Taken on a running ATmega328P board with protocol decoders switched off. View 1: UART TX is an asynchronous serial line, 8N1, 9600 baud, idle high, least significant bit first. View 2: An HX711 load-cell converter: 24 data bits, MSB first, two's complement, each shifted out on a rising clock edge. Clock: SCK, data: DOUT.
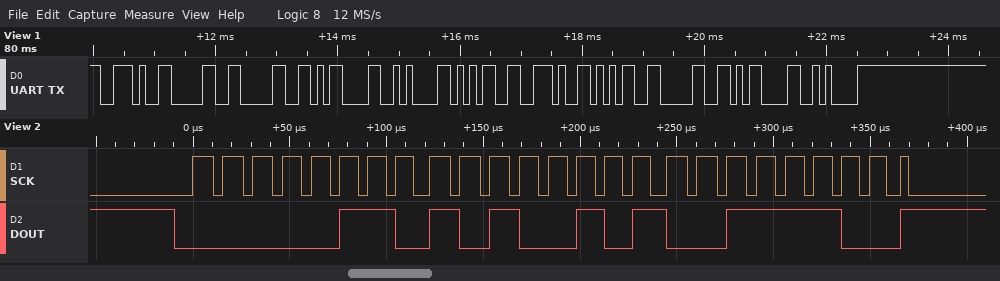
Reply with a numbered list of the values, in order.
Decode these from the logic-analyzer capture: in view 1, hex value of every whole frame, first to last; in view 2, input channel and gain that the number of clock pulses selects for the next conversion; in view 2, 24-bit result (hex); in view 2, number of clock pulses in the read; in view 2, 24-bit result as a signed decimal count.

1. 2E 30 30 0D 0A 35 2E 35 30 0D 0A
2. channel A, gain 128
3. 0x06A53C
4. 25
5. 435516
